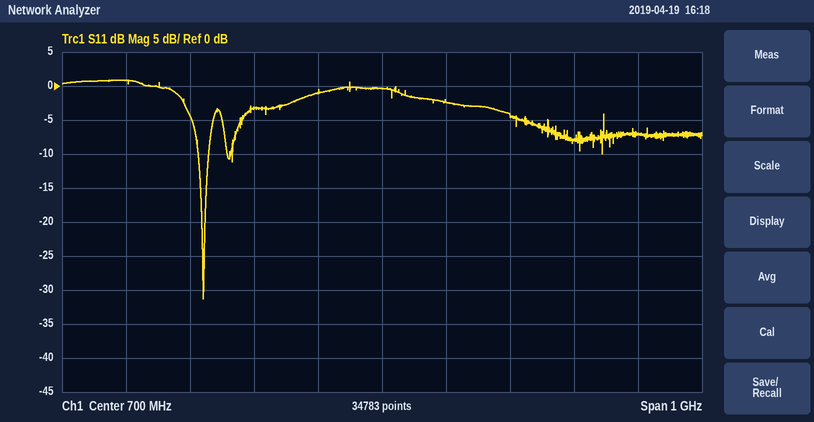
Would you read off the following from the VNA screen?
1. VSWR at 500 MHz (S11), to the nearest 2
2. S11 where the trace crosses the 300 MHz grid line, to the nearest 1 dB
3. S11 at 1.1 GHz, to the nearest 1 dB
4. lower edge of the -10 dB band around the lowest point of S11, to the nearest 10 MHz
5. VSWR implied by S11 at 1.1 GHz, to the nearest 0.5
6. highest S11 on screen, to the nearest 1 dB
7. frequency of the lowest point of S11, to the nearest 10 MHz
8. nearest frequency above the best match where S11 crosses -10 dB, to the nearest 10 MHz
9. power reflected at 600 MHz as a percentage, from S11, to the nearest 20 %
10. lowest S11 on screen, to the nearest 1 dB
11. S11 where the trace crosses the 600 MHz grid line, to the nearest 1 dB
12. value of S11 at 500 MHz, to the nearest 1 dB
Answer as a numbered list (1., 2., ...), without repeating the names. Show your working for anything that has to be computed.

1. |Γ| = 10^(-3/20) = 0.7079; VSWR = (1 + 0.7079)/(1 − 0.7079) ≈ 6
2. 1 dB
3. -7 dB
4. 410 MHz
5. |Γ| = 10^(-7/20) = 0.4467; VSWR = (1 + 0.4467)/(1 − 0.4467) ≈ 2.61, so 2.5 to the nearest 0.5
6. 1 dB
7. 420 MHz
8. 430 MHz
9. 10^(-1/10) ≈ 79.4 %, so 80 % to the nearest 20 %
10. -31 dB
11. -1 dB
12. -3 dB
